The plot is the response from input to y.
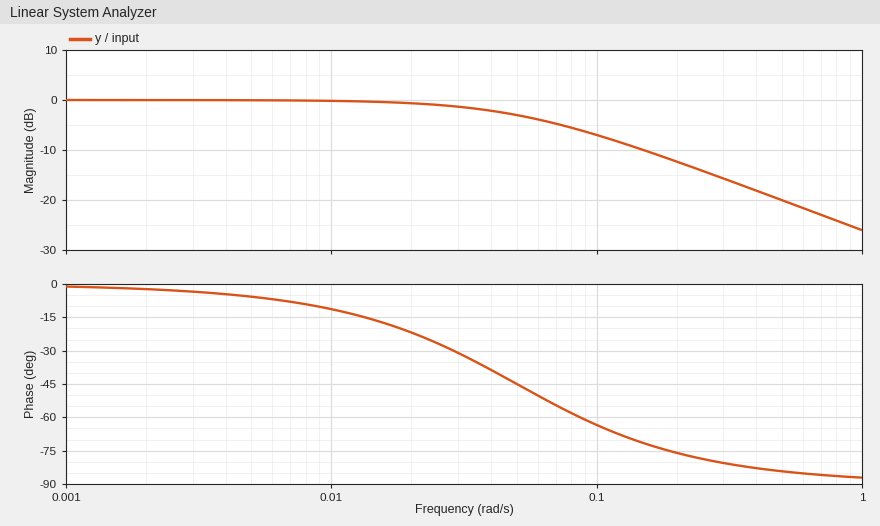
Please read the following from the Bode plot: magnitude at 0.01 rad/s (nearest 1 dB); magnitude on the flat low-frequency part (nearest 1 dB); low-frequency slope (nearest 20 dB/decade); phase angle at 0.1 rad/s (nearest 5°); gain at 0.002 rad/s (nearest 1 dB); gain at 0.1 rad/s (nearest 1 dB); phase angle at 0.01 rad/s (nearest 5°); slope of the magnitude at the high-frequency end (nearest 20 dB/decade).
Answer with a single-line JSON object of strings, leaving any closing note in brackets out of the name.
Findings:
{"magnitude at 0.01 rad/s": "0 dB", "magnitude on the flat low-frequency part": "0 dB", "low-frequency slope": "0 dB/decade", "phase angle at 0.1 rad/s": "-65°", "gain at 0.002 rad/s": "0 dB", "gain at 0.1 rad/s": "-7 dB", "phase angle at 0.01 rad/s": "-10°", "slope of the magnitude at the high-frequency end": "-20 dB/decade"}
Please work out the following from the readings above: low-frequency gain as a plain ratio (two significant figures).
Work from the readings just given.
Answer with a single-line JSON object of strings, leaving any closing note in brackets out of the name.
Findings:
{"low-frequency gain as a plain ratio": "1.0"}
